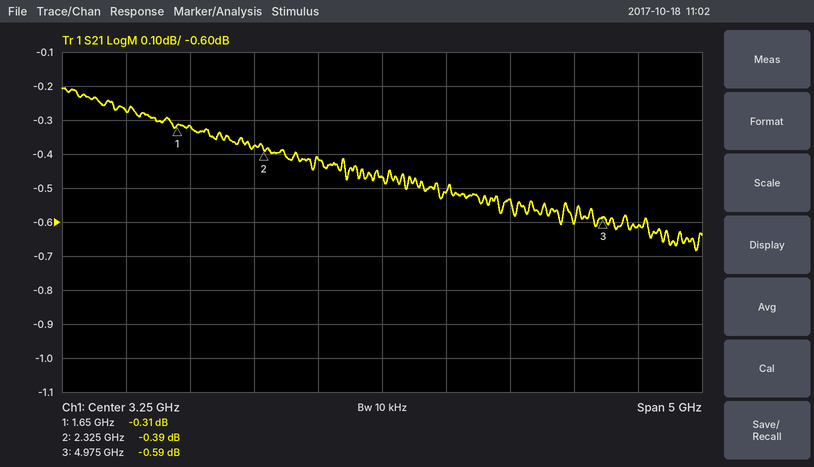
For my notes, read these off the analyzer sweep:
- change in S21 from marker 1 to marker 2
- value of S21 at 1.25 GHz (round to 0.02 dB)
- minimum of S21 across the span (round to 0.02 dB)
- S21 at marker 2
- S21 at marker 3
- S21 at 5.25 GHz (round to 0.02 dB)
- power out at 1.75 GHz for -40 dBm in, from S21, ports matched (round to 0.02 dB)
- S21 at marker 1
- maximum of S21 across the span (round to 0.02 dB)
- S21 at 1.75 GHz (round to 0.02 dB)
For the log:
-0.08 dB
-0.28 dB
-0.68 dB
-0.39 dB
-0.59 dB
-0.62 dB
-40.32 dBm
-0.31 dB
-0.20 dB
-0.32 dB
